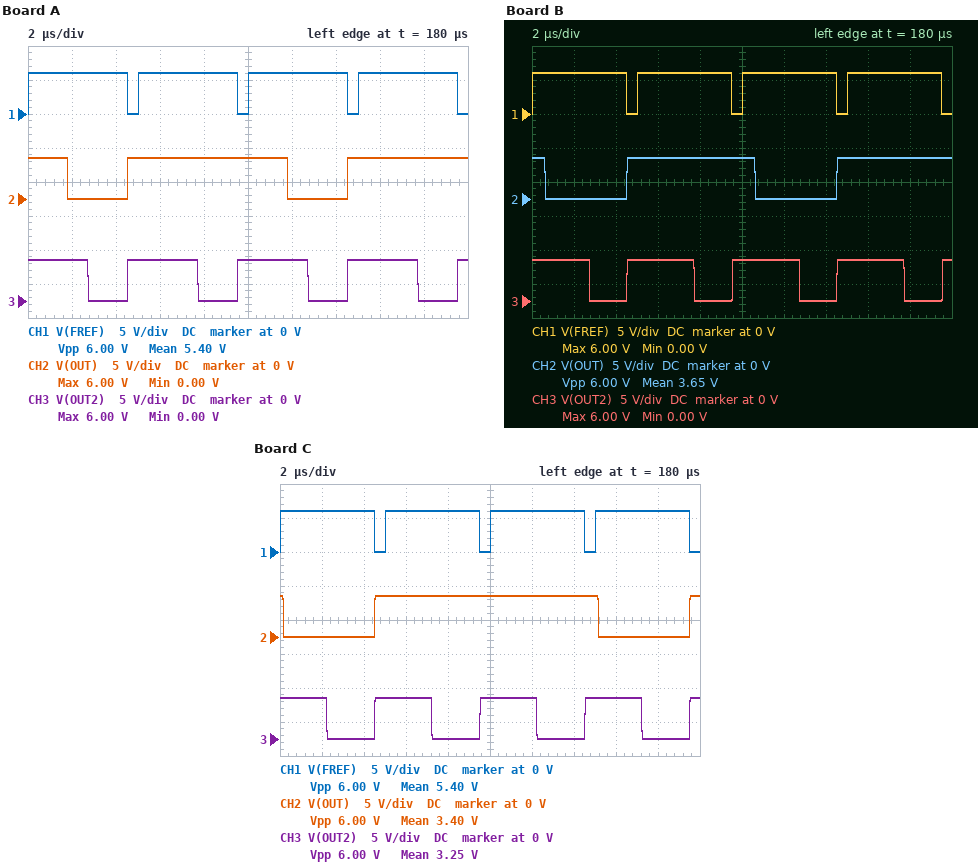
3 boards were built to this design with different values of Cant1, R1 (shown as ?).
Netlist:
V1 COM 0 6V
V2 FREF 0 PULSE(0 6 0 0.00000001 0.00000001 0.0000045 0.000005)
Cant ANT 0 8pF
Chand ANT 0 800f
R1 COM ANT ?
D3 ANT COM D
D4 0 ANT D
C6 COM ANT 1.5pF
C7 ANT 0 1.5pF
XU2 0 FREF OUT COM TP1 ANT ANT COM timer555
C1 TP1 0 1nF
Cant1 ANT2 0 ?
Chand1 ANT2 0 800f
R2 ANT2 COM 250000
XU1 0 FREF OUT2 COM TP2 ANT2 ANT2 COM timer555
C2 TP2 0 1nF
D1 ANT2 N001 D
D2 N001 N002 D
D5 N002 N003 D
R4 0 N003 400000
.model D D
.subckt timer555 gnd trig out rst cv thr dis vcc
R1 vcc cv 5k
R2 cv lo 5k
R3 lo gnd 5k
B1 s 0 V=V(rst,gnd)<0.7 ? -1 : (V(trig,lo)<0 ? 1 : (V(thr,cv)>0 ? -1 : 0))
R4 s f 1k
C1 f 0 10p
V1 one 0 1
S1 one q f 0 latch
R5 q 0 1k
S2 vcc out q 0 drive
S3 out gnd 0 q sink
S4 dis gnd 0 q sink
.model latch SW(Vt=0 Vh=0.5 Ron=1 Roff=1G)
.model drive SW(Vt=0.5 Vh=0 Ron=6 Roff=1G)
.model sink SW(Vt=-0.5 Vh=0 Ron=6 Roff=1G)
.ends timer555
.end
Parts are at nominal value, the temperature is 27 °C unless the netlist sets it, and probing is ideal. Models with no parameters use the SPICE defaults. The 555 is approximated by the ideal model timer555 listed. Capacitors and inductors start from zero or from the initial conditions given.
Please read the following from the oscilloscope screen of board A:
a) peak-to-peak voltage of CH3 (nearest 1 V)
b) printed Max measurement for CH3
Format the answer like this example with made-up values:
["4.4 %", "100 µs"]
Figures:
["6 V", "6.00 V"]
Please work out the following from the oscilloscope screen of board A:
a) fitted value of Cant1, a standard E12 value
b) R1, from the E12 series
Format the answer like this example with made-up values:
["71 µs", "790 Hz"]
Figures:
["6.8 pF", "560 kΩ"]
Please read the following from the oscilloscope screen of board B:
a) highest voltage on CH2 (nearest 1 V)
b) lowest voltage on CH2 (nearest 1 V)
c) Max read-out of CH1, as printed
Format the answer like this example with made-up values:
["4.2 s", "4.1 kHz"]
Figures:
["6 V", "0 V", "6.00 V"]
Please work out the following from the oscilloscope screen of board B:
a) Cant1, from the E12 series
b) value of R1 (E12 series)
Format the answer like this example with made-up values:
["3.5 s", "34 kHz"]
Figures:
["6.8 pF", "470 kΩ"]
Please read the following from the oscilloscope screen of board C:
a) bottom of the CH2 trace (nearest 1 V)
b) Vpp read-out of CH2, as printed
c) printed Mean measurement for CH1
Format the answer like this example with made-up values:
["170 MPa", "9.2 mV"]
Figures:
["0 V", "6.00 V", "5.40 V"]
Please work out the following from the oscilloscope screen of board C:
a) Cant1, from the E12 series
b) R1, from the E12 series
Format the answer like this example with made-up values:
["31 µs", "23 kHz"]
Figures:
["5.6 pF", "820 kΩ"]
